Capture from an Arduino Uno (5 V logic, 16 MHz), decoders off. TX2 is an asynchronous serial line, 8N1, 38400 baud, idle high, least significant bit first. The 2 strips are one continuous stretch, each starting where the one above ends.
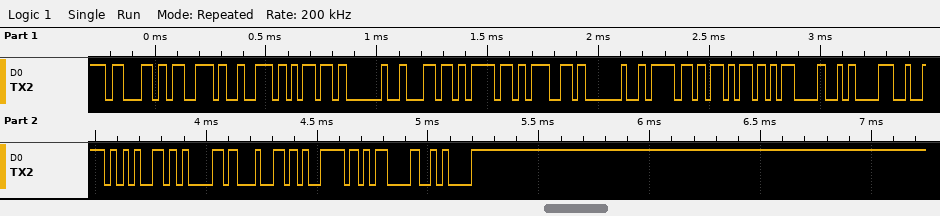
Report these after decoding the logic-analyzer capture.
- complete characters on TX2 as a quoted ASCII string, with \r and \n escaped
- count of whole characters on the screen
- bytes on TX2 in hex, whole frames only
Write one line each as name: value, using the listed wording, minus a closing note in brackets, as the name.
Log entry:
complete characters on TX2 as a quoted ASCII string, with \r and \n escaped: "csrm log ok\r\nready\r\n"
count of whole characters on the screen: 20
bytes on TX2 in hex, whole frames only: 0x63 0x73 0x72 0x6D 0x20 0x6C 0x6F 0x67 0x20 0x6F 0x6B 0x0D 0x0A 0x72 0x65 0x61 0x64 0x79 0x0D 0x0A
